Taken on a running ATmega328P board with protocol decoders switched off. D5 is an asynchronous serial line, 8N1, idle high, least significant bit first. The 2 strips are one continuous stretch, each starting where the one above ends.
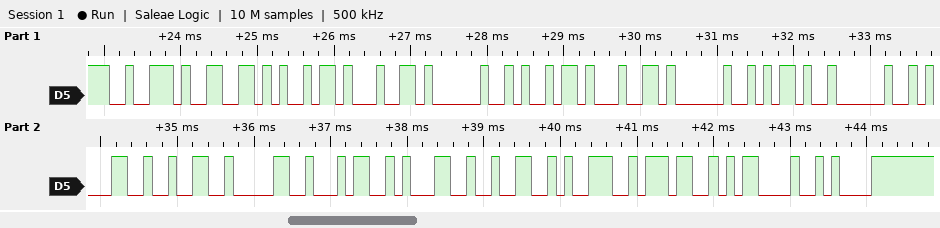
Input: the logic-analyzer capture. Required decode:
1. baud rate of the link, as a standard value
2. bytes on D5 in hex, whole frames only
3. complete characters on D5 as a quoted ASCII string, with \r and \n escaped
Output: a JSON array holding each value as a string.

["9600 baud", "72 66 69 64 20 69 64 20 2D 20 31 32 30 34 31 32 39 37 0D 0A", "\"rfid id - 12041297\\r\\n\""]
